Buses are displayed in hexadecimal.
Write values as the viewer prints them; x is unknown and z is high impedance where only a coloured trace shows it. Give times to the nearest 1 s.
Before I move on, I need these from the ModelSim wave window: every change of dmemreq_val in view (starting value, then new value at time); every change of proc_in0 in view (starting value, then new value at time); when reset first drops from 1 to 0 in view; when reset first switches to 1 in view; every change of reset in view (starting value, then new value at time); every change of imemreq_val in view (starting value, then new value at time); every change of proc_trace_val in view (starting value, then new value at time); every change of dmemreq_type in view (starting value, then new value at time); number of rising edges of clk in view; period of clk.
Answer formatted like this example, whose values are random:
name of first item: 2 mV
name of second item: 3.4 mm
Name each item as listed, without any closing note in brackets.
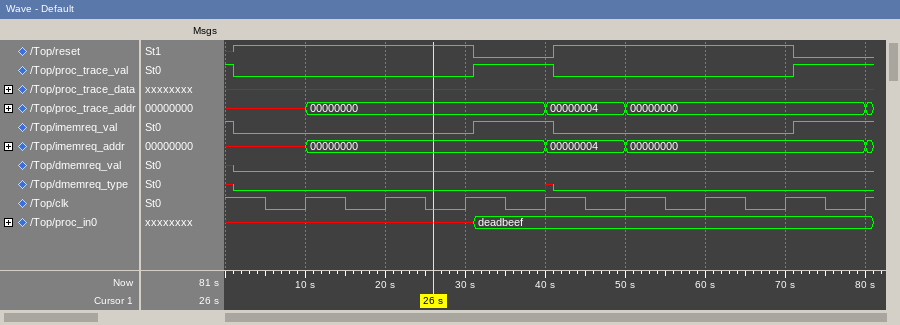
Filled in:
every change of dmemreq_val in view: x, 0 at 1 s
every change of proc_in0 in view: x, deadbeef at 31 s
when reset first drops from 1 to 0 in view: 31 s
when reset first switches to 1 in view: 1 s
every change of reset in view: x, 1 at 1 s, 0 at 31 s, 1 at 41 s, 0 at 71 s
every change of imemreq_val in view: 1, 0 at 1 s, 1 at 31 s, 0 at 41 s, 1 at 71 s
every change of proc_trace_val in view: 1, 0 at 1 s, 1 at 31 s, 0 at 41 s, 1 at 71 s
every change of dmemreq_type in view: x, 0 at 1 s, x at 40 s, 0 at 41 s
number of rising edges of clk in view: 8
period of clk: 10 s
